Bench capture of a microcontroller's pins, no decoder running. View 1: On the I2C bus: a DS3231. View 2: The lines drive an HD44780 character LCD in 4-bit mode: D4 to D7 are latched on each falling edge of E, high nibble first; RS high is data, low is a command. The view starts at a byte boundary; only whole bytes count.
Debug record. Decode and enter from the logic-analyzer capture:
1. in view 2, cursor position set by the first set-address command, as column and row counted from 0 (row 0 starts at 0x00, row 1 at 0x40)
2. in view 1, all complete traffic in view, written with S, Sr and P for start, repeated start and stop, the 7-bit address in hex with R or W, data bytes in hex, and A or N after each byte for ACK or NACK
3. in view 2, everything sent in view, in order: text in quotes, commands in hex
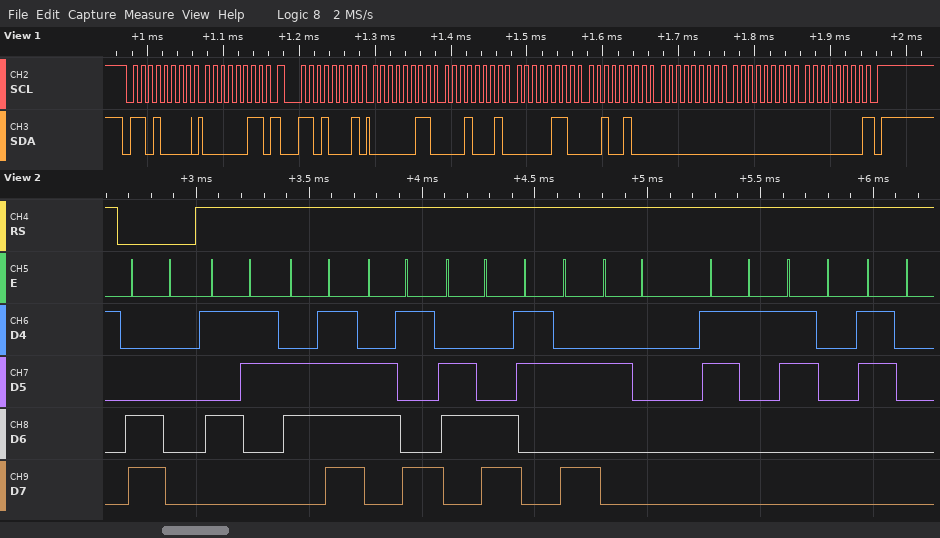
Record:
column 0, row 1
S 68W A 03 A Sr 68R A 03 A 11 A 06 A 24 A 00 A 00 A 00 N P
0xC0 "Soil: 100"
